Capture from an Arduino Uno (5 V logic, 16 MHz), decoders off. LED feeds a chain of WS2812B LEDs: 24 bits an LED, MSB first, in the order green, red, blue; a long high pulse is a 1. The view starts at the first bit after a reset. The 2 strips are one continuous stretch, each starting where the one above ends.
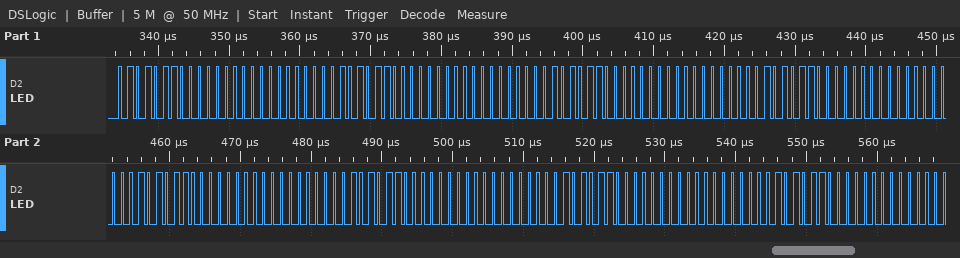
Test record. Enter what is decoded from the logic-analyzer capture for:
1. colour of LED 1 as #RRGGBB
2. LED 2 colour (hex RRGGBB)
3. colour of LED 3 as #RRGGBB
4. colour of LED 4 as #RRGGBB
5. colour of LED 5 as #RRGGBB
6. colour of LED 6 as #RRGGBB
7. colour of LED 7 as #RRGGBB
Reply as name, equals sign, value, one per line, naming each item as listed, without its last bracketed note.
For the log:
colour of LED 1 as #RRGGBB = #005600
LED 2 colour = #005600
colour of LED 3 as #RRGGBB = #005600
colour of LED 4 as #RRGGBB = #005600
colour of LED 5 as #RRGGBB = #005600
colour of LED 6 as #RRGGBB = #005600
colour of LED 7 as #RRGGBB = #005600
